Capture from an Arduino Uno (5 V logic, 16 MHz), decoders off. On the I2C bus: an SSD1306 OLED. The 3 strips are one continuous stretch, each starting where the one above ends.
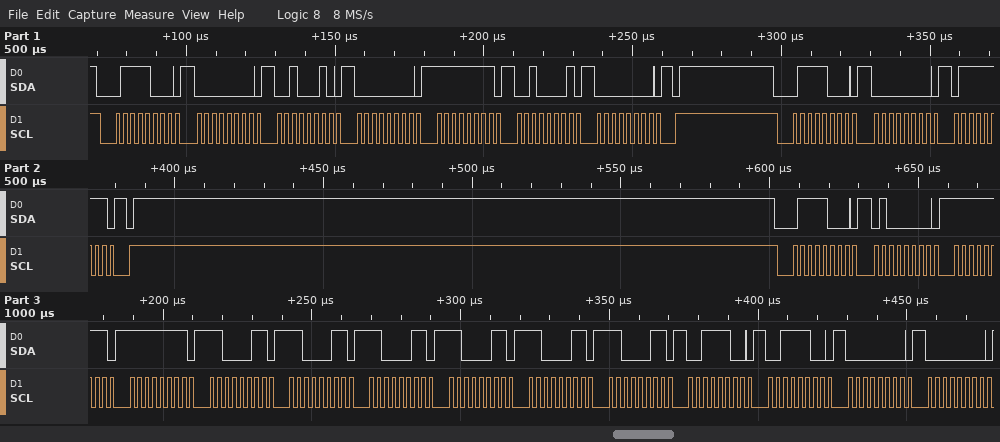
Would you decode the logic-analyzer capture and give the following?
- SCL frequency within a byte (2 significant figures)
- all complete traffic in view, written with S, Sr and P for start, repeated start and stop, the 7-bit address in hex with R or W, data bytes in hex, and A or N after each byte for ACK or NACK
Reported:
400 kHz
S 3CW A 00 A 22 A 00 A FF A 21 A 00 A P S 3CW A 00 A 7F A P S 3CW A 40 A FF A FF A C3 A C3 A C3 A C3 A C3 A C3 A 3C A 3C A 00 A 00 A
